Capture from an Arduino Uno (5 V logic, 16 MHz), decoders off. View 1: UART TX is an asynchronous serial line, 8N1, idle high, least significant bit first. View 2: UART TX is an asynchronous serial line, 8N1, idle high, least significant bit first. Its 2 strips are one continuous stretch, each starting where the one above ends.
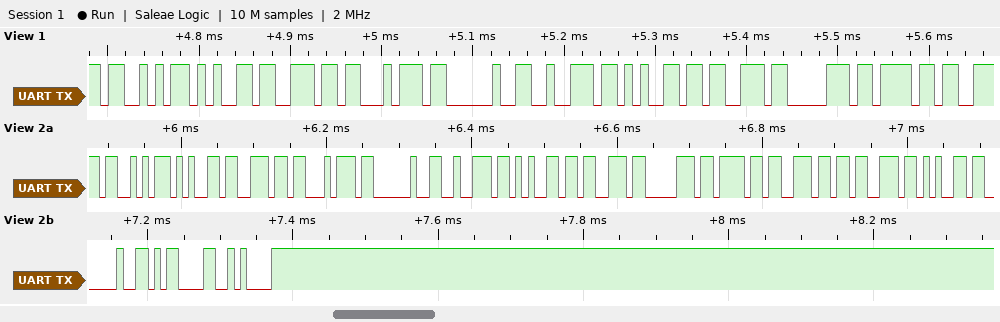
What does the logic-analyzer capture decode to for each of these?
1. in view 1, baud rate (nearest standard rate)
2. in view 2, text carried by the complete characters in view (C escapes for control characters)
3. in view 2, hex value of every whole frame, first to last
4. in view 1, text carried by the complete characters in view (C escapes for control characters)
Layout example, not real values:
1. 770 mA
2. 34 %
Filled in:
1. 115200 baud
2. "Sent response \r\n"
3. 53 65 6E 74 20 72 65 73 70 6F 6E 73 65 20 0D 0A
4. "Sent respo"
